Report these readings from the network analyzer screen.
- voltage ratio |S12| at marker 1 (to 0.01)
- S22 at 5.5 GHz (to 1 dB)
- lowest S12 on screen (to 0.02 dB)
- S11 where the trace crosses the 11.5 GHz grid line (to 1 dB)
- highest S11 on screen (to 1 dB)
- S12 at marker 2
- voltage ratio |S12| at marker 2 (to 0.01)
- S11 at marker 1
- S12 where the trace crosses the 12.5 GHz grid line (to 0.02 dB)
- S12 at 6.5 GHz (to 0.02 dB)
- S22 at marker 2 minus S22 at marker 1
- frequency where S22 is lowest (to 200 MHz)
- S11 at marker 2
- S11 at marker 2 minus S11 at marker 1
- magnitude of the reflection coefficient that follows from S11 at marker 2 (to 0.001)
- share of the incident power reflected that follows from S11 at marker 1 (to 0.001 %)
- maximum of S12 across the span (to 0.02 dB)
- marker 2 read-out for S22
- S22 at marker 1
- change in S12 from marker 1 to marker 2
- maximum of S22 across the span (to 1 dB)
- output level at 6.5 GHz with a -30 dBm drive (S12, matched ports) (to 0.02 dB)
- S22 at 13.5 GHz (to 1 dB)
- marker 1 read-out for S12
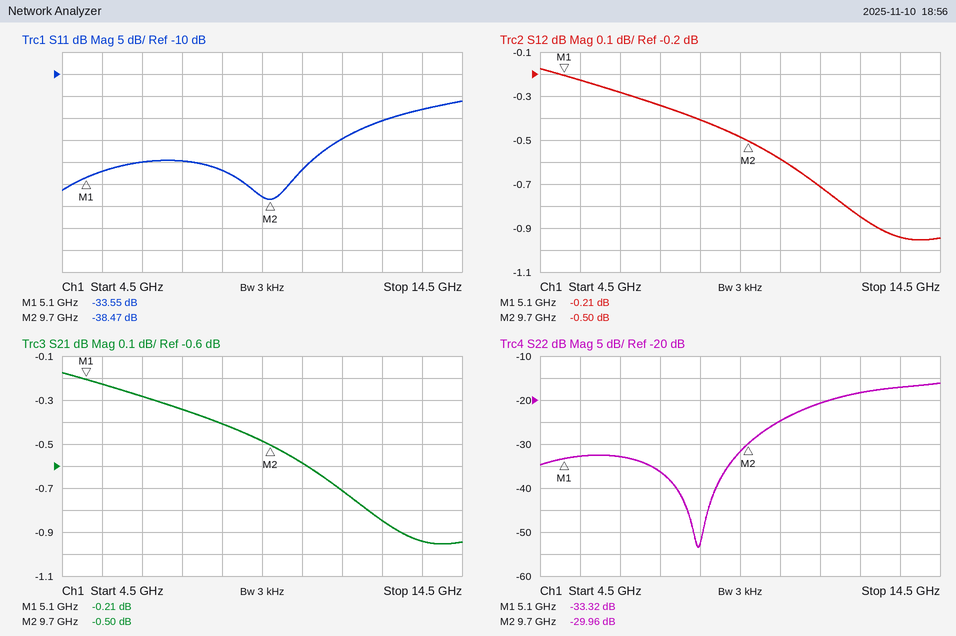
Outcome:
0.98
-33 dB
-0.96 dB
-25 dB
-16 dB
-0.50 dB
0.94
-33.55 dB
-0.84 dB
-0.28 dB
3.36 dB
8.4 GHz
-38.47 dB
-4.92 dB
0.012
0.044 %
-0.18 dB
-29.96 dB
-33.32 dB
-0.29 dB
-16 dB
-30.28 dBm
-17 dB
-0.21 dB
